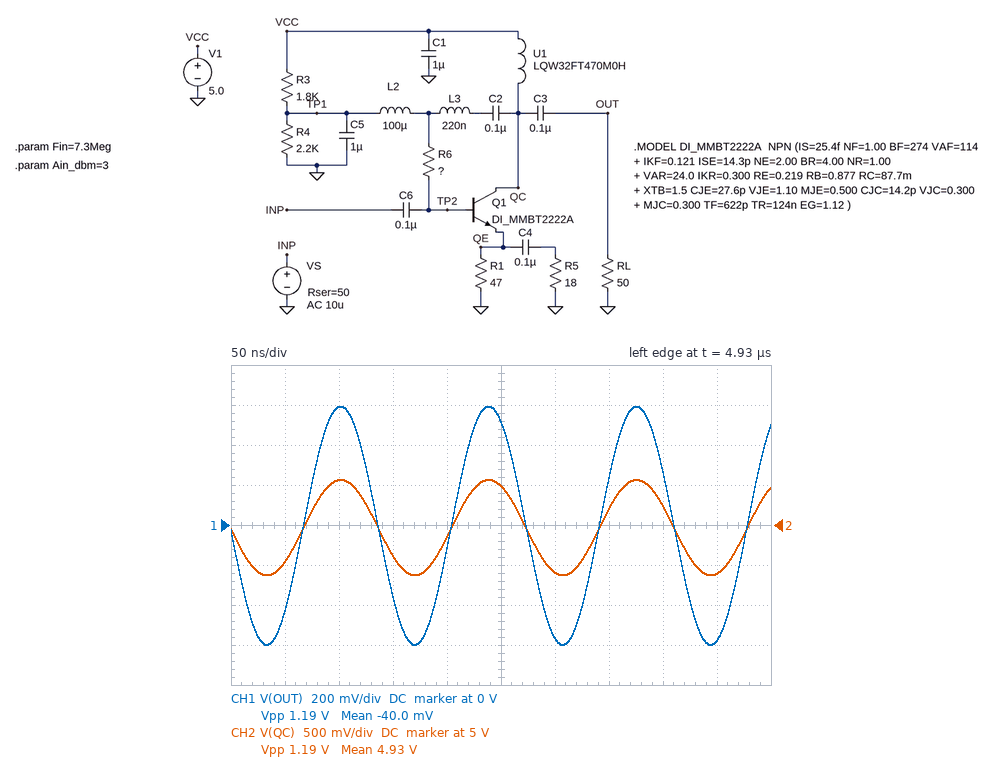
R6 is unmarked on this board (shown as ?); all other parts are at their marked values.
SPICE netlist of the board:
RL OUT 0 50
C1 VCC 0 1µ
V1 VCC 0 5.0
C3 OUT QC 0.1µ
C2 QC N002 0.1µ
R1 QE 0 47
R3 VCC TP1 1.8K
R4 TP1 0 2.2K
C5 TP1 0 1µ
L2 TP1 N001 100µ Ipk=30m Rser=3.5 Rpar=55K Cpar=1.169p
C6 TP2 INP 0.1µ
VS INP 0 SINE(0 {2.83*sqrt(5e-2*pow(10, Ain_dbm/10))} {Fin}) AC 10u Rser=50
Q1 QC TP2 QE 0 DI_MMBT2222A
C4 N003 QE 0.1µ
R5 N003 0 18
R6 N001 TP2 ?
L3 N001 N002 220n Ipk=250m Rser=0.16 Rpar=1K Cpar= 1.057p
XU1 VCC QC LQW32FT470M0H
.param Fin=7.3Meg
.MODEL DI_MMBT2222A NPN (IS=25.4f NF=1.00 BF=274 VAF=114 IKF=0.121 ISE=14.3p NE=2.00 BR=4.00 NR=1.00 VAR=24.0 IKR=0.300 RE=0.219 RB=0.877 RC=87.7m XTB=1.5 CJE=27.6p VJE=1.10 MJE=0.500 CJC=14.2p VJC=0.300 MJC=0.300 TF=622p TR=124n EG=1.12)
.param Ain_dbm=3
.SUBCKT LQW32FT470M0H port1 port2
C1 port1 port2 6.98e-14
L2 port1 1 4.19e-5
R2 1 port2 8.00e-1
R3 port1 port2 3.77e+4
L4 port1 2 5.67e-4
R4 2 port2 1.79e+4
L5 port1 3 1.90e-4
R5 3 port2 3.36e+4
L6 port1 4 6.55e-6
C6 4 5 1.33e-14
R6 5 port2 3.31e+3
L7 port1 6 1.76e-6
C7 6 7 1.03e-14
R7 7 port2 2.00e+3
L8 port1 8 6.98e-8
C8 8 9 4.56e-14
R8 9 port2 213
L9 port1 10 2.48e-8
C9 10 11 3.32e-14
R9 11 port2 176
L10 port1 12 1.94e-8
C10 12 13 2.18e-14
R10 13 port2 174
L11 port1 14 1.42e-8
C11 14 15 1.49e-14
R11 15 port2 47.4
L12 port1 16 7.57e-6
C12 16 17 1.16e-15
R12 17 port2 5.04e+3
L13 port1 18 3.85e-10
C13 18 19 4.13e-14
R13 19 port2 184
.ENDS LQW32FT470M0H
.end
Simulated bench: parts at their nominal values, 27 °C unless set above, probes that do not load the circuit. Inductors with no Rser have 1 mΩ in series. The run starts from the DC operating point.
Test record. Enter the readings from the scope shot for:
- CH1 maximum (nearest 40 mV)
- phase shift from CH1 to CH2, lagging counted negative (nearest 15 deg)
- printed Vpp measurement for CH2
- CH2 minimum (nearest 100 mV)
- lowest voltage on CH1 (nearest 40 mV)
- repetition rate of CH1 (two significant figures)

600 mV
0 deg
1.19 V
4.4 V
-600 mV
7.3 MHz
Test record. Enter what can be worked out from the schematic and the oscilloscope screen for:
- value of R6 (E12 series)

82 Ω
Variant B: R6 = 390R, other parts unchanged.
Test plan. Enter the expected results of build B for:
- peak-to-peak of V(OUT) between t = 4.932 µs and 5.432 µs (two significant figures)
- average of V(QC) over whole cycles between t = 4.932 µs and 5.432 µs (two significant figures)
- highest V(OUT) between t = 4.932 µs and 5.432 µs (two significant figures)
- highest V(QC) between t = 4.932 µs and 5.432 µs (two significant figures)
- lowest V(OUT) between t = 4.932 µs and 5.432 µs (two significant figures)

3.3 V
5.0 V
1.6 V
6.5 V
-1.7 V
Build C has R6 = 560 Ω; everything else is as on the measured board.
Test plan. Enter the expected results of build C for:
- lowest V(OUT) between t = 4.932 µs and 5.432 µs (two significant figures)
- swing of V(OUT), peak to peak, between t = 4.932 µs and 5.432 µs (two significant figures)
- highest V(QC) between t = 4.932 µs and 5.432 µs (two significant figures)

-1.9 V
3.6 V
6.6 V
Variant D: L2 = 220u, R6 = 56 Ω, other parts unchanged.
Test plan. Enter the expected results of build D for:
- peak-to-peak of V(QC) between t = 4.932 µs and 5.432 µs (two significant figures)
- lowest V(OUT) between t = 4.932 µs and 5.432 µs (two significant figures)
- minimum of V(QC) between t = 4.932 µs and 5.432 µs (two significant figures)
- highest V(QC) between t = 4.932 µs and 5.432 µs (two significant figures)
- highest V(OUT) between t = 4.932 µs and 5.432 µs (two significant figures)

810 mV
-410 mV
4.6 V
5.4 V
400 mV
